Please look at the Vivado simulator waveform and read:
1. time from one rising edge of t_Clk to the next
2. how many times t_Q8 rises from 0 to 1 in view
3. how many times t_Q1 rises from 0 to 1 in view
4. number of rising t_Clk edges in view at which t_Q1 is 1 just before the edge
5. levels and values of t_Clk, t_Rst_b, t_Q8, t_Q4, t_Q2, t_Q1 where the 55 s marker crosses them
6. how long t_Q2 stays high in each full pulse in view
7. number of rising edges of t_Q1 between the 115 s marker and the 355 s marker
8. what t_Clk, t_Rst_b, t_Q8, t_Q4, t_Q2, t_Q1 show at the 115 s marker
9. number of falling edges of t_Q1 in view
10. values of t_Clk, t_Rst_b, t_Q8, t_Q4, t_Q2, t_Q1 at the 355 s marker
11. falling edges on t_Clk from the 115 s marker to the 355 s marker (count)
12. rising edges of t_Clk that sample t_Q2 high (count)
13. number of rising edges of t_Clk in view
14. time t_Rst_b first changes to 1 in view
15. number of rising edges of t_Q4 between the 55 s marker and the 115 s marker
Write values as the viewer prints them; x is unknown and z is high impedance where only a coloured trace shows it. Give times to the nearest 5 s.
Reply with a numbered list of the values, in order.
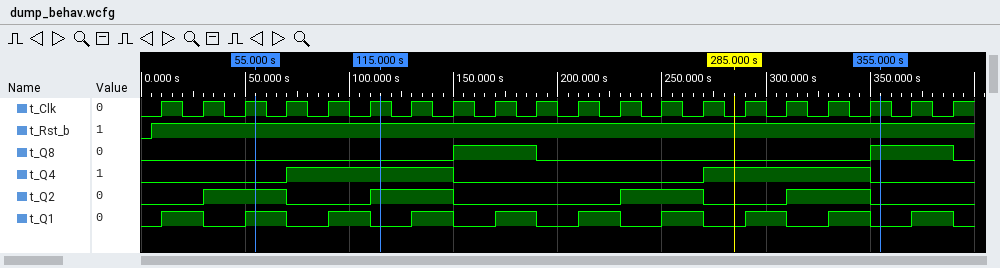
1. 20 s
2. 2
3. 10
4. 10
5. t_Clk=1, t_Rst_b=1, t_Q8=0, t_Q4=0, t_Q2=1, t_Q1=1
6. 40 s, 40 s, 40 s, 40 s
7. 6
8. t_Clk=1, t_Rst_b=1, t_Q8=0, t_Q4=1, t_Q2=1, t_Q1=0
9. 10
10. t_Clk=1, t_Rst_b=1, t_Q8=1, t_Q4=0, t_Q2=0, t_Q1=0
11. 12
12. 8
13. 20
14. 5 s
15. 1
